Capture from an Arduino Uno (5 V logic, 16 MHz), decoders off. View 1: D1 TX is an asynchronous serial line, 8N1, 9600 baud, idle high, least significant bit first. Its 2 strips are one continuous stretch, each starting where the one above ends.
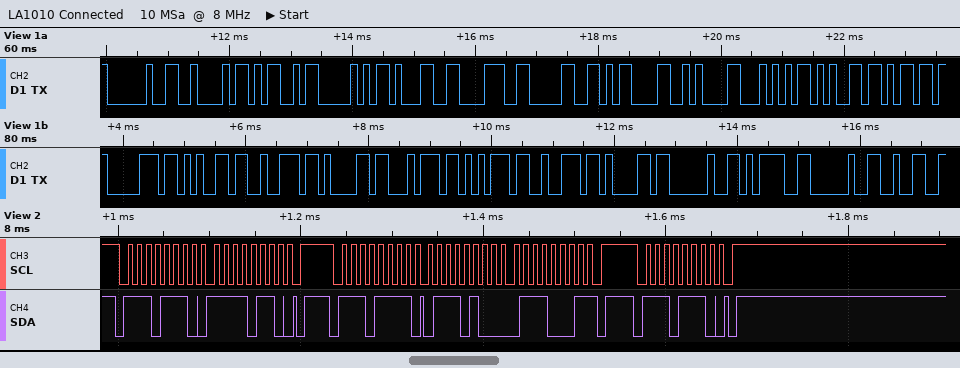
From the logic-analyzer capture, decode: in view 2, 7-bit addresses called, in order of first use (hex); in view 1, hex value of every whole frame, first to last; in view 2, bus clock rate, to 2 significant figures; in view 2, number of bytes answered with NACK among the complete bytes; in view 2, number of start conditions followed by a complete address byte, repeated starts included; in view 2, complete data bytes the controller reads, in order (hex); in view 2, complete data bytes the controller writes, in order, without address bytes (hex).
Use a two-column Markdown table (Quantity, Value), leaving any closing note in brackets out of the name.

| Quantity | Value |
|---|---|
| in view 2, 7-bit addresses called, in order of first use | 0x77 |
| in view 1, hex value of every whole frame, first to last | 20 42 4D 50 31 38 30 0D 0A 54 65 6D 70 65 72 61 74 75 72 61 20 3D 20 32 |
| in view 2, bus clock rate, to 2 significant figures | 100 kHz |
| in view 2, number of bytes answered with NACK among the complete bytes | 1 |
| in view 2, number of start conditions followed by a complete address byte, repeated starts included | 3 |
| in view 2, complete data bytes the controller reads, in order | 74 71 |
| in view 2, complete data bytes the controller writes, in order, without address bytes | F6 |
